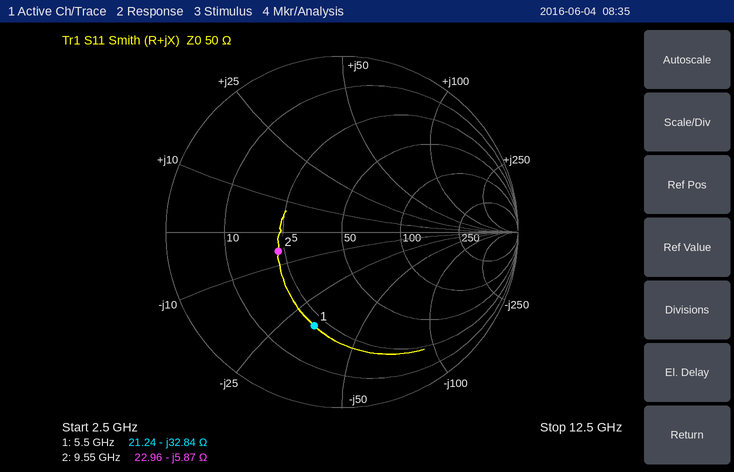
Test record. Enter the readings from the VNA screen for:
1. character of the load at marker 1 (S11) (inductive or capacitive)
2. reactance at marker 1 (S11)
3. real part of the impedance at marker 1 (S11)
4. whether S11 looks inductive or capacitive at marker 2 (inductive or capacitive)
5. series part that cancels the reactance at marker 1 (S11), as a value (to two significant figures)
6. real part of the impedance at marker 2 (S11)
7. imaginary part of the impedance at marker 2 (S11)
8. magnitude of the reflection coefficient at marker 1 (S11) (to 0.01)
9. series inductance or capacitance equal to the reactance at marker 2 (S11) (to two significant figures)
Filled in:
capacitive
-32.84 Ω
21.24 Ω
capacitive
950 pH
22.96 Ω
-5.87 Ω
0.56
2.8 pF
